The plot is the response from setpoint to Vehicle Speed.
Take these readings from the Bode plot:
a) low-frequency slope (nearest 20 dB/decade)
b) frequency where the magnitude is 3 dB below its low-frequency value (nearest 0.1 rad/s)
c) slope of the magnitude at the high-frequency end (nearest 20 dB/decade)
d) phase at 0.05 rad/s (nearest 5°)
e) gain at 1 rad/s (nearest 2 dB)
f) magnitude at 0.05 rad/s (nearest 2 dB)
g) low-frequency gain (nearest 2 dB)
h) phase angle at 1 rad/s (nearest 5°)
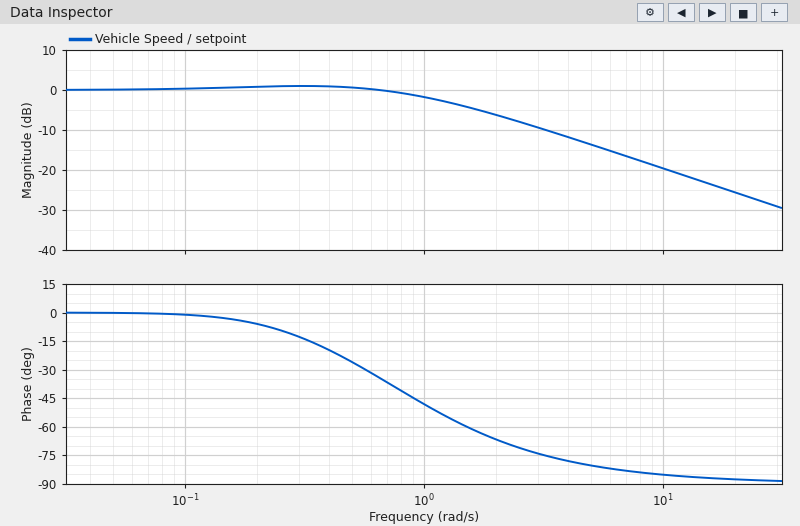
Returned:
0 dB/decade
1.2 rad/s
-20 dB/decade
0°
-2 dB
0 dB
0 dB
-50°
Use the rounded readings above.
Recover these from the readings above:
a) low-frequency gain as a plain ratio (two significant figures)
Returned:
1.0
